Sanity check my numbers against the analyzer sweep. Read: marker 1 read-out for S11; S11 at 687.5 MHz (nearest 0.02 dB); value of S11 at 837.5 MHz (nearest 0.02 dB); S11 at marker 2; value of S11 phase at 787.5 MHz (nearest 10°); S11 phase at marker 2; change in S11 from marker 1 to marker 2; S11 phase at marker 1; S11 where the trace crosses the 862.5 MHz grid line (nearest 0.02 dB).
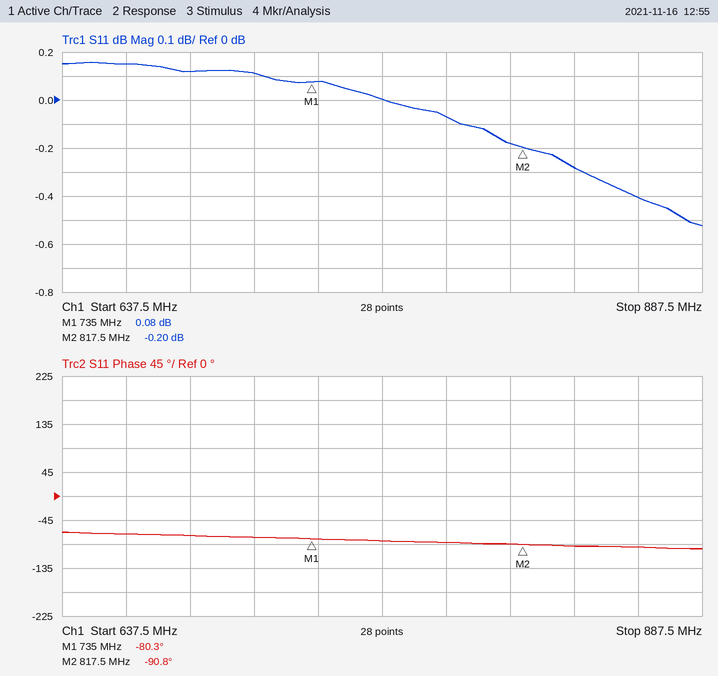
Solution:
0.08 dB
0.12 dB
-0.28 dB
-0.20 dB
-90°
-90.8°
-0.28 dB
-80.3°
-0.40 dB
